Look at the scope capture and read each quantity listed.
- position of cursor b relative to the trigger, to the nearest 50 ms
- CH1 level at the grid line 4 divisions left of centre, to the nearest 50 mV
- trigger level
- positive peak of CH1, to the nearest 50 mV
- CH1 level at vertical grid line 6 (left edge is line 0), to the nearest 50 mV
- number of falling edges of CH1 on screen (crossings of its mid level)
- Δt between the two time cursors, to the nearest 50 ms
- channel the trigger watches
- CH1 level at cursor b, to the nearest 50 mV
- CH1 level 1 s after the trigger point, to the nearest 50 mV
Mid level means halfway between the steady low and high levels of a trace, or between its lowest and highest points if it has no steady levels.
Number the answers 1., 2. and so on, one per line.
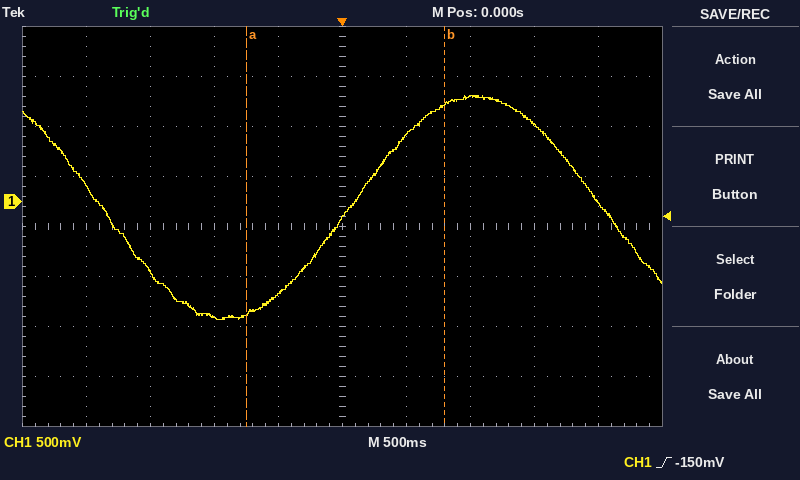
1. +800 ms
2. 150 mV
3. -150 mV
4. 1.05 V
5. 650 mV
6. 2
7. 1.55 s
8. CH1
9. 950 mV
10. 1.05 V
